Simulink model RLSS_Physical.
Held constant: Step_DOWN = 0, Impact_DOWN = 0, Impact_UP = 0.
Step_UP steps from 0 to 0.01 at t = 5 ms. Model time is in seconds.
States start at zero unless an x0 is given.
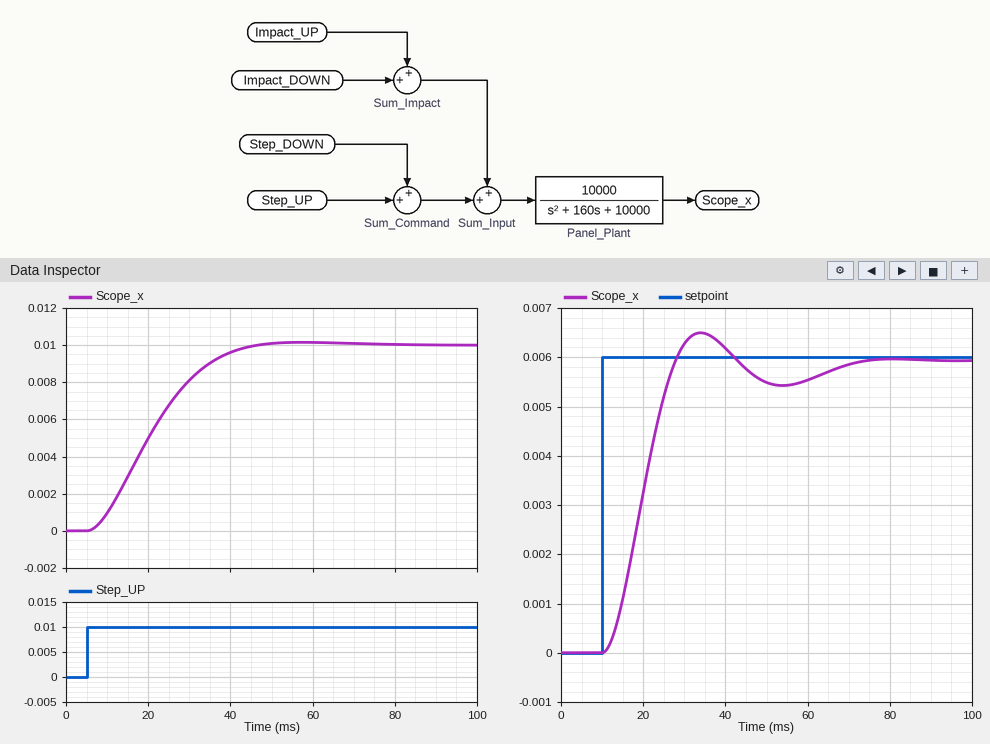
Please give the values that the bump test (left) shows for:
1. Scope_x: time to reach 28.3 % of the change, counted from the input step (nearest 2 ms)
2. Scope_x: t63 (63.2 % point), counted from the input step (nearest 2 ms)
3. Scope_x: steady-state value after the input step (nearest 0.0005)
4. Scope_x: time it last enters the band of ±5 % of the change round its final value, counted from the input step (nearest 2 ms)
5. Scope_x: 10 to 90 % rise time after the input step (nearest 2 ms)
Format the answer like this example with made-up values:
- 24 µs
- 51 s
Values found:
- 10 ms
- 18 ms
- 0.0100
- 34 ms
- 24 ms
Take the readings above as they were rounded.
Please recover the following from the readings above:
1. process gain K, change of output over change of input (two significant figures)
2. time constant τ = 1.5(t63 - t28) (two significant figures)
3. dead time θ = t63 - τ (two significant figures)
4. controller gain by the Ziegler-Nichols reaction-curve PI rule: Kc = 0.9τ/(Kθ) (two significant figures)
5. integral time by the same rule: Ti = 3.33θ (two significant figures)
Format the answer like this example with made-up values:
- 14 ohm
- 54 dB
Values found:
- 1.0
- 12 ms
- 6.0 ms
- 1.8
- 20 ms
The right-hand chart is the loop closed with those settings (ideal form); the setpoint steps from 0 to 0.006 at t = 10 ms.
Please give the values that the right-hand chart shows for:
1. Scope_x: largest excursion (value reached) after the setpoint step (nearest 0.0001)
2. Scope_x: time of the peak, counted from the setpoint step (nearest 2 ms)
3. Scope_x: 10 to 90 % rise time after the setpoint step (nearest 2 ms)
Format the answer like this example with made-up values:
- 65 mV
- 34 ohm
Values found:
- 0.0065
- 24 ms
- 12 ms
